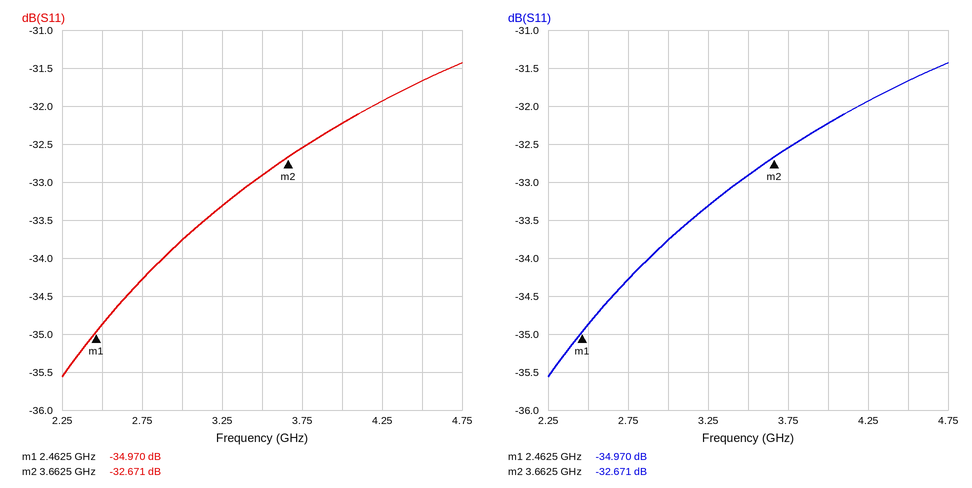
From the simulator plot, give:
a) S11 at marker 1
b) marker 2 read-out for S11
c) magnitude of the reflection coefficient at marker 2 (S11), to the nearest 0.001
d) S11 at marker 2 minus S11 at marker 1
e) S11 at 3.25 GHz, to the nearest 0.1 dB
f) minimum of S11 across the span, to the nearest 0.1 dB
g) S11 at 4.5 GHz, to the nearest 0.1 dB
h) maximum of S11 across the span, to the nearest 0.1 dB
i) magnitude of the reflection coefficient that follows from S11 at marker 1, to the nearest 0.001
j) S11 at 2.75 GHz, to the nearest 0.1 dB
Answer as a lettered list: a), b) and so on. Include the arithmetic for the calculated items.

a) -34.970 dB
b) -32.671 dB
c) 10^(-32.671/20) ≈ 0.023
d) -32.671 − (-34.97) = 2.299 dB
e) -33.3 dB
f) -35.6 dB
g) -31.7 dB
h) -31.4 dB
i) 10^(-34.97/20) ≈ 0.018
j) -34.3 dB
